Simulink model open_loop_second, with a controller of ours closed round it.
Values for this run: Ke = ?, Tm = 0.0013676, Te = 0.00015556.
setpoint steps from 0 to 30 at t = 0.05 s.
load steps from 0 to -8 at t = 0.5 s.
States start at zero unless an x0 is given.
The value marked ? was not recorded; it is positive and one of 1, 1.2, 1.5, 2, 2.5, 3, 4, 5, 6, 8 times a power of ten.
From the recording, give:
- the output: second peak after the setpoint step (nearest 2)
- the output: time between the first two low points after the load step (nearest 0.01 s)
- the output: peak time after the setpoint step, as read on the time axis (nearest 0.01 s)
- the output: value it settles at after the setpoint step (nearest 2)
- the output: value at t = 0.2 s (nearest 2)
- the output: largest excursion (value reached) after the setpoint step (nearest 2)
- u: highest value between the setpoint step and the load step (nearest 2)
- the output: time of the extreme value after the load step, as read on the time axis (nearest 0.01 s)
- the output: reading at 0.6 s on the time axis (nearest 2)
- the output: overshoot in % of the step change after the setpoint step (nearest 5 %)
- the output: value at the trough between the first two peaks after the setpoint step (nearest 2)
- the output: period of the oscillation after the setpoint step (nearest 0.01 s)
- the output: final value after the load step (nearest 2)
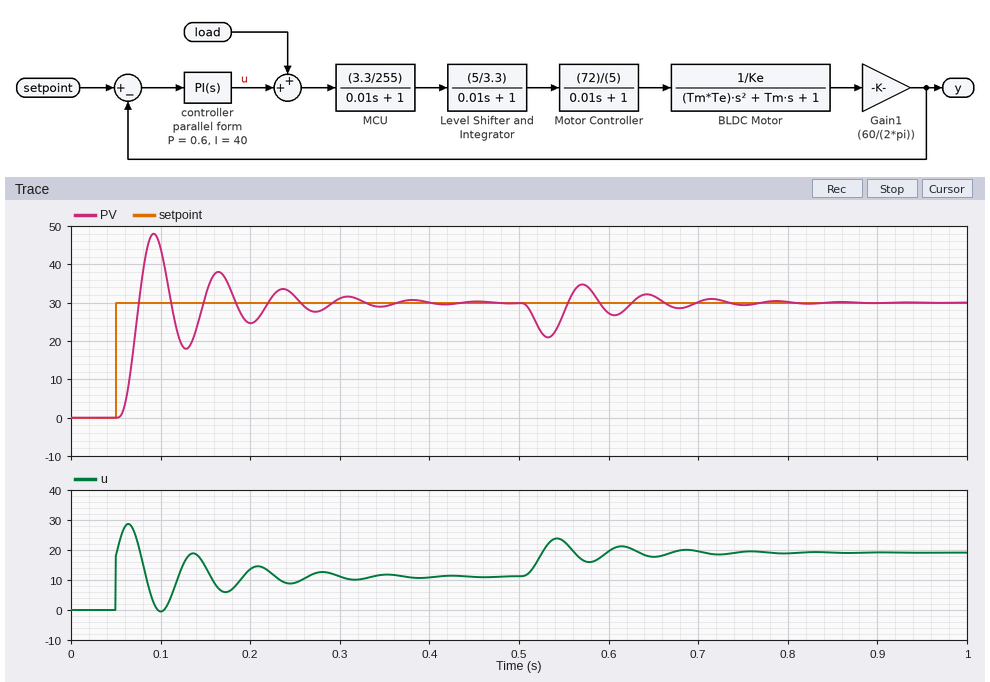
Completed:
38
0.07 s
0.09 s
30
24
48
28
0.53 s
28
60 %
18
0.07 s
30
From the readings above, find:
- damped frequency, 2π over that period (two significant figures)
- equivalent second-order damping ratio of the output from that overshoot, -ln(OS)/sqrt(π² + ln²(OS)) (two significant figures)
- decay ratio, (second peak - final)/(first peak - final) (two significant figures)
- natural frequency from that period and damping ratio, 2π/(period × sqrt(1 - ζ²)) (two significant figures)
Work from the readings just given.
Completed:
90 rad/s
0.16
0.44
91 rad/s
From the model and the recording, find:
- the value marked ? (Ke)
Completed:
1
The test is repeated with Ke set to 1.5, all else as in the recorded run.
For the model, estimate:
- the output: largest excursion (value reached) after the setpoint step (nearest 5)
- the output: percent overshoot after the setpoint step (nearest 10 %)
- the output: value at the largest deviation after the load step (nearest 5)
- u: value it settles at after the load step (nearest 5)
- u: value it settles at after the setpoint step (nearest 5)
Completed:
40
40 %
25
25
15
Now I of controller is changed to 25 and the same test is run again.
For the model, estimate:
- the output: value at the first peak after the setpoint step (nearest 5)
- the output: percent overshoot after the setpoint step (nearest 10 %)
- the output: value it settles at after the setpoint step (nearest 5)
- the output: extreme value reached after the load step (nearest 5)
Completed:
40
30 %
30
20
